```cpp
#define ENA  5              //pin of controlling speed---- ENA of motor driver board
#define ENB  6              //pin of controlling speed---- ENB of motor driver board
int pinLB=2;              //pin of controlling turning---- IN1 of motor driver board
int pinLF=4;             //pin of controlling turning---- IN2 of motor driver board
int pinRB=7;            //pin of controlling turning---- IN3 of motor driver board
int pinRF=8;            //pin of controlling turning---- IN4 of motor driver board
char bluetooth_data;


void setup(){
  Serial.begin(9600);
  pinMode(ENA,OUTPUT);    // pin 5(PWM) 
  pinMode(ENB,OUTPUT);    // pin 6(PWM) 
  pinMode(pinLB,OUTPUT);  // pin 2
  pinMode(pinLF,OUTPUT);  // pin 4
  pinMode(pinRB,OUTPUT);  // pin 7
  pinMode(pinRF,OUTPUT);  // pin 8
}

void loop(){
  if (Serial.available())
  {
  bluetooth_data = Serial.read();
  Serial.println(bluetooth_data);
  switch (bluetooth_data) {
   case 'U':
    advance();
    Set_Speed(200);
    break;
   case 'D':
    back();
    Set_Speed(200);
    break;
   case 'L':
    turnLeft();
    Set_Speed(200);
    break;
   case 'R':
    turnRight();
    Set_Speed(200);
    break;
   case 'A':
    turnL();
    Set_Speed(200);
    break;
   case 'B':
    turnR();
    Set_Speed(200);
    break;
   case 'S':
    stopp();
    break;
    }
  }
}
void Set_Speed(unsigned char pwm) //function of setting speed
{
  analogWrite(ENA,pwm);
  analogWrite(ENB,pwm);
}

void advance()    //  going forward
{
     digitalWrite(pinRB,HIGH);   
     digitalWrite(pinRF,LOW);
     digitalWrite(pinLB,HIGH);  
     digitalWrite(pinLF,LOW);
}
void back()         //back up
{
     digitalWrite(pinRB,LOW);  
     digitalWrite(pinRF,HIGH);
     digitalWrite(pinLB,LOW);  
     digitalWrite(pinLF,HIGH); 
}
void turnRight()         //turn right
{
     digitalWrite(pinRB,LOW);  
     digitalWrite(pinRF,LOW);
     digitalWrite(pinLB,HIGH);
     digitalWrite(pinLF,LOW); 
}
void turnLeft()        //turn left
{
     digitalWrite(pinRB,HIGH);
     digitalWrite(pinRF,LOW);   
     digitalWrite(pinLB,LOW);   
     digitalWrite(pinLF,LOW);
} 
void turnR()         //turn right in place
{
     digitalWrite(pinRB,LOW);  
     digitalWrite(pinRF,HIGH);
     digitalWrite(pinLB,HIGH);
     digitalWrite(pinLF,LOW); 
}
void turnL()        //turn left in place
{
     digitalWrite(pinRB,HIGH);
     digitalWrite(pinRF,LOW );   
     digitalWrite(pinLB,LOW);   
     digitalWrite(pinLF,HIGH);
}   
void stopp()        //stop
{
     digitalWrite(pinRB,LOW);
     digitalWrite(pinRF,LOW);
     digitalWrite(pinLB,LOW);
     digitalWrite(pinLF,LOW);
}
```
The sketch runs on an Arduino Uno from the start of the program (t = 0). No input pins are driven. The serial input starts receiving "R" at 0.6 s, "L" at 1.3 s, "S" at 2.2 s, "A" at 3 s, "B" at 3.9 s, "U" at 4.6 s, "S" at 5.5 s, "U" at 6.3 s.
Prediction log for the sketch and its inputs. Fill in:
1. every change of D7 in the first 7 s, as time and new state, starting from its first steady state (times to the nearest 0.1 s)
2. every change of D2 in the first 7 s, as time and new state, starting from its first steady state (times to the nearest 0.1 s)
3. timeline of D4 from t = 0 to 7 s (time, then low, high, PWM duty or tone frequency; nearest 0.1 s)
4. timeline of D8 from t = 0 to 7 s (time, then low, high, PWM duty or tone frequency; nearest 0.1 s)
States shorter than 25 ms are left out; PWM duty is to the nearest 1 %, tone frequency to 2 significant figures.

0 s low; 1.3 s high; 2.2 s low; 3 s high; 3.9 s low; 4.6 s high; 5.5 s low; 6.3 s high
0 s low; 0.6 s high; 1.3 s low; 3.9 s high; 5.5 s low; 6.3 s high
0 s low; 3 s high; 3.9 s low
0 s low; 3.9 s high; 4.6 s low
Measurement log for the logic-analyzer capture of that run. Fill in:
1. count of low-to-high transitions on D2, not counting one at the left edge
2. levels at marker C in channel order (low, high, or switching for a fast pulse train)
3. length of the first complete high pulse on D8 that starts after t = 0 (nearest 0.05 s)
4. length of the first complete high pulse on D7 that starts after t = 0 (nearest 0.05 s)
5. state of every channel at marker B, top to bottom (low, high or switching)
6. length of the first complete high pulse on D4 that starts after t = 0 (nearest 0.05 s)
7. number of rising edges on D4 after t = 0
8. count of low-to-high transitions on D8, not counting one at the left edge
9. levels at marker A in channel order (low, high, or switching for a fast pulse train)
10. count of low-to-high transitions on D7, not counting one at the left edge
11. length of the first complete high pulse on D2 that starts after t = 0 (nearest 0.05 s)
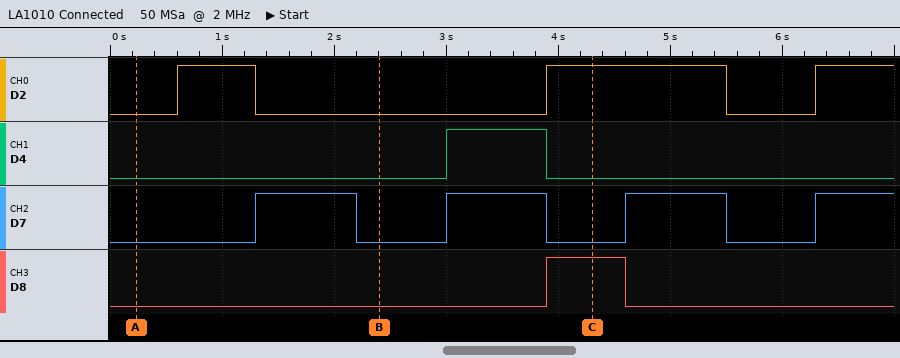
3
D2 high, D4 low, D7 low, D8 high
0.70 s
0.90 s
D2 low, D4 low, D7 low, D8 low
0.90 s
1
1
D2 low, D4 low, D7 low, D8 low
4
0.70 s
